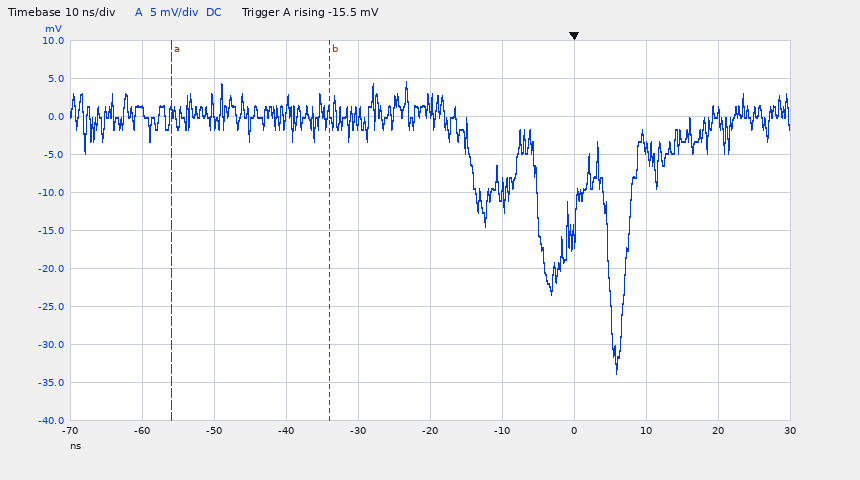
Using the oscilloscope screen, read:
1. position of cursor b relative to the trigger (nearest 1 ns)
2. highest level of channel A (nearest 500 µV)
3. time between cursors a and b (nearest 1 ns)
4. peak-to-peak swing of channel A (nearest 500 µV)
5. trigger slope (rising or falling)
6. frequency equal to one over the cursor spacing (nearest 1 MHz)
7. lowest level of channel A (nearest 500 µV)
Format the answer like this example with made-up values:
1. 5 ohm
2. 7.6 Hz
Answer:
1. -34 ns
2. 4.5 mV
3. 22 ns
4. 38.5 mV
5. rising
6. 45 MHz
7. -34.0 mV
